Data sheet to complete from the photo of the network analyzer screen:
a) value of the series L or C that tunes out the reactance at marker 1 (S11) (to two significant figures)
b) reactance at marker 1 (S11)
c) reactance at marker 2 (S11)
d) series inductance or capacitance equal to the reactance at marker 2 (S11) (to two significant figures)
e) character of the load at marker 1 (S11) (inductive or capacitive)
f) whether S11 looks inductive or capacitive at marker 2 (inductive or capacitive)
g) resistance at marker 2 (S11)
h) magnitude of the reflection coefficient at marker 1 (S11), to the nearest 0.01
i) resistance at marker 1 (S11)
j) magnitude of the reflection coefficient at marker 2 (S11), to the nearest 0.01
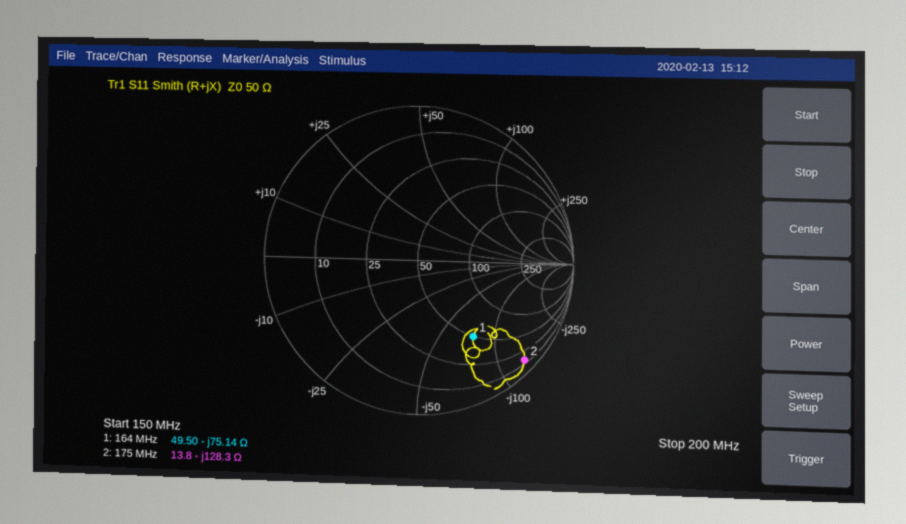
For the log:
73 nH
-75.14 Ω
-128.3 Ω
7.1 pF
capacitive
capacitive
13.8 Ω
0.60
49.50 Ω
0.93
